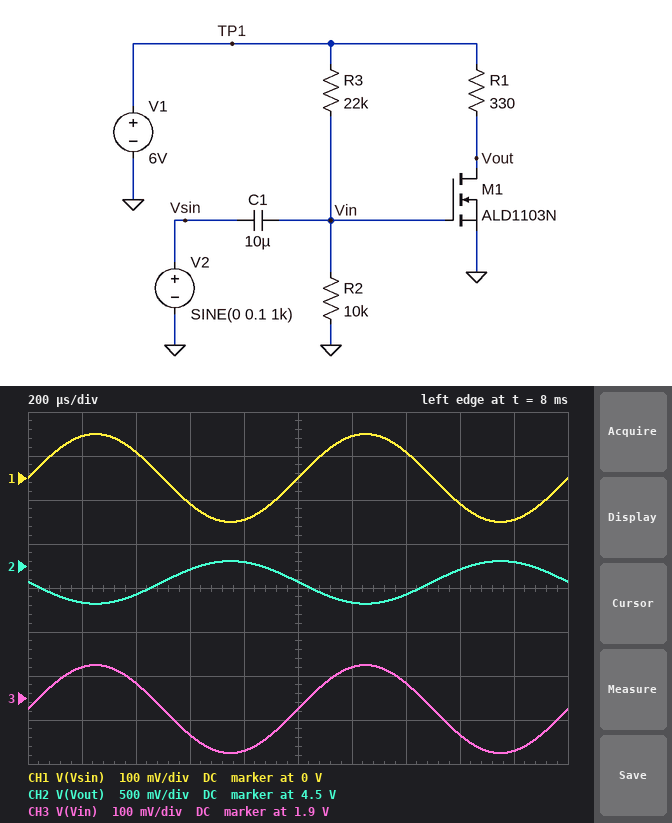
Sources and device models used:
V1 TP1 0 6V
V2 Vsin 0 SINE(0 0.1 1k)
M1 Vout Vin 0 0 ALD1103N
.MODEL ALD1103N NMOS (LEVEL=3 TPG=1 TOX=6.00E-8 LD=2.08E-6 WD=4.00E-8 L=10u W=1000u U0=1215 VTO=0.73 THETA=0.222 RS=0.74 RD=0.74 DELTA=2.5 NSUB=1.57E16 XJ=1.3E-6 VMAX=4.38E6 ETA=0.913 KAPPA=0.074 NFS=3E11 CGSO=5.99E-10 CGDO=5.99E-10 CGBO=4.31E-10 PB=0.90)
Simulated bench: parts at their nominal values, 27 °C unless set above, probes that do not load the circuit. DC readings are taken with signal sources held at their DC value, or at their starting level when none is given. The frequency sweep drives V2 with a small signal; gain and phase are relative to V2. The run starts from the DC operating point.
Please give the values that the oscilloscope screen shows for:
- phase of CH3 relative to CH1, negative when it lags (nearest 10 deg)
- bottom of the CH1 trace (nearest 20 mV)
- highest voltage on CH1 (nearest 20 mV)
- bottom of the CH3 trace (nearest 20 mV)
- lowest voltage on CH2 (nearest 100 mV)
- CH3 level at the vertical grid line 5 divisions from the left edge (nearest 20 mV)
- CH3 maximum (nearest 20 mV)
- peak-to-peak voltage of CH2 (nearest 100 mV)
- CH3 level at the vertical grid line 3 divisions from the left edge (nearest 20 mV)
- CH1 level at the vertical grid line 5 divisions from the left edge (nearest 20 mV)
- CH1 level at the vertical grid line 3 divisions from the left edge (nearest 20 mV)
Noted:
0 deg
-100 mV
100 mV
1.78 V
4.1 V
1.88 V
1.98 V
500 mV
1.82 V
0 V
-60 mV
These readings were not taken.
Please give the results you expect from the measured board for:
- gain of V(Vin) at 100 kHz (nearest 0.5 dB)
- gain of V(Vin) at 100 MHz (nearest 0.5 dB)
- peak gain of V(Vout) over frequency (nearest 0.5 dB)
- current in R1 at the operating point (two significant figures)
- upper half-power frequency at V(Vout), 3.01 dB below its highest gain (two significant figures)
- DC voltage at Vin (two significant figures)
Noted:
0 dB
0 dB
7.5 dB
5.1 mA
1.0 GHz
1.9 V
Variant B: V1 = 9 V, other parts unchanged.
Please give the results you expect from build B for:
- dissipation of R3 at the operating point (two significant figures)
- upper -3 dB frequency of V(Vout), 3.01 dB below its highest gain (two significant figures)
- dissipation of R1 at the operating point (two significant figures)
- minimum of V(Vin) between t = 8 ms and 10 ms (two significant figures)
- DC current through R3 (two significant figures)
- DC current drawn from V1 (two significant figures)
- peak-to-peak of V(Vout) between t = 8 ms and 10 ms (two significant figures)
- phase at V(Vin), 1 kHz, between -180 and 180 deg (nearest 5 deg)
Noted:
1.7 mW
910 MHz
62 mW
2.7 V
280 µA
14 mA
680 mV
0 deg
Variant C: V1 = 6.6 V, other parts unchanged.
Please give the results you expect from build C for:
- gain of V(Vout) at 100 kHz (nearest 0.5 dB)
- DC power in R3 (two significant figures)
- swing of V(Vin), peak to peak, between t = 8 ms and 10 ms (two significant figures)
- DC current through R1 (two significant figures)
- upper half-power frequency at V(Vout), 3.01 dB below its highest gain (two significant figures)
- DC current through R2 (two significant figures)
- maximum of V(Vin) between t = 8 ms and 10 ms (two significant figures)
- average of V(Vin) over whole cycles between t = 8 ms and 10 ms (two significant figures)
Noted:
8.5 dB
940 µW
200 mV
6.6 mA
980 MHz
210 µA
2.2 V
2.1 V
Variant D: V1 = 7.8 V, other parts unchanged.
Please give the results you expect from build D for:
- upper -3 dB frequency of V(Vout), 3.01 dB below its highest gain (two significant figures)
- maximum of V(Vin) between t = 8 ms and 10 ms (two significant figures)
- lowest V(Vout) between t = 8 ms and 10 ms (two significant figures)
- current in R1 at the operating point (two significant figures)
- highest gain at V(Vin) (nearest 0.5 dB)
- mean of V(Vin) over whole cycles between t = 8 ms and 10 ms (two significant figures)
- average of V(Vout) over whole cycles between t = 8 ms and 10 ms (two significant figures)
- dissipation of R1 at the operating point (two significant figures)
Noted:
940 MHz
2.5 V
4.2 V
9.9 mA
0 dB
2.4 V
4.5 V
32 mW
